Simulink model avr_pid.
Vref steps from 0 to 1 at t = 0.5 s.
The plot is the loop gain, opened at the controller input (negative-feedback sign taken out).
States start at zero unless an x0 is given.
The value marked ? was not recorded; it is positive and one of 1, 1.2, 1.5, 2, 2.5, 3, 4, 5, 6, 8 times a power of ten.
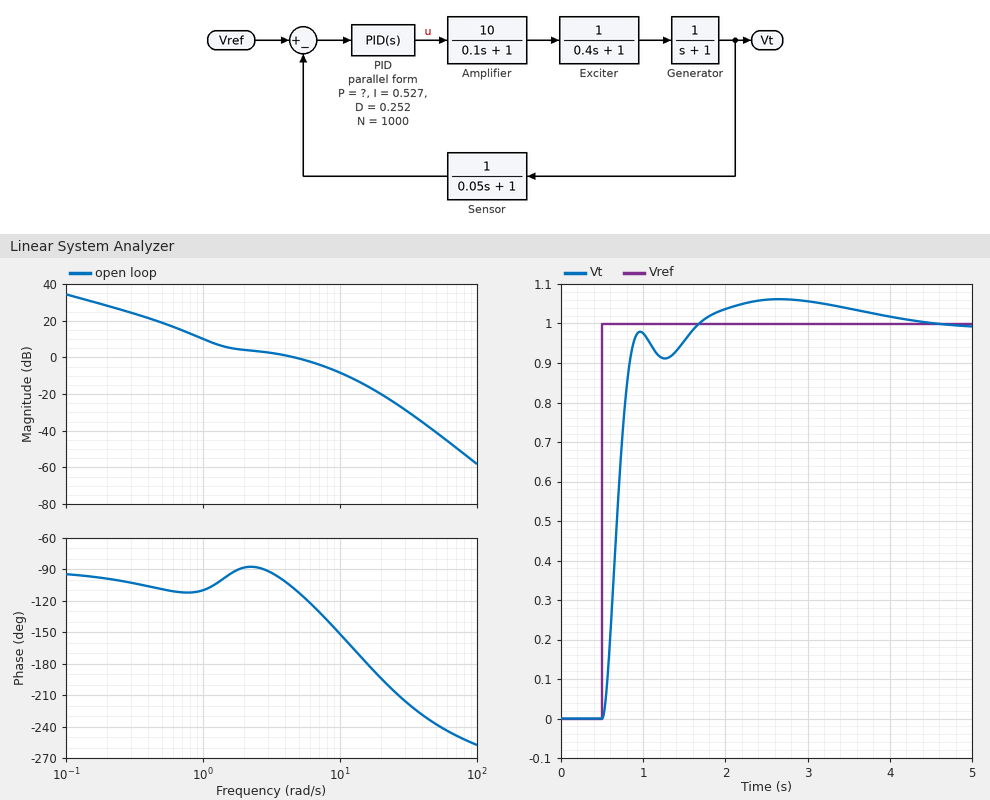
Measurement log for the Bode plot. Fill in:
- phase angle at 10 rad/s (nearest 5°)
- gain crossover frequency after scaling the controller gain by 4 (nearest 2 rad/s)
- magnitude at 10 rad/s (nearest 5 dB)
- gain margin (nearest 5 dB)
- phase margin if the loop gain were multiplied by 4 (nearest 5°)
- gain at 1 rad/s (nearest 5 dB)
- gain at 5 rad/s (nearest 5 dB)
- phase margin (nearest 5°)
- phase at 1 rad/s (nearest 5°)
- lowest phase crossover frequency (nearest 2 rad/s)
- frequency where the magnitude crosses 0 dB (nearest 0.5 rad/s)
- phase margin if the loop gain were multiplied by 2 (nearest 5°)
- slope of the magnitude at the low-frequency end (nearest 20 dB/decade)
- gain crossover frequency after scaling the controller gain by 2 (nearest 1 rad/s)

-150°
12 rad/s
-10 dB
15 dB
15°
10 dB
0 dB
70°
-110°
16 rad/s
4.5 rad/s
40°
-20 dB/decade
8 rad/s
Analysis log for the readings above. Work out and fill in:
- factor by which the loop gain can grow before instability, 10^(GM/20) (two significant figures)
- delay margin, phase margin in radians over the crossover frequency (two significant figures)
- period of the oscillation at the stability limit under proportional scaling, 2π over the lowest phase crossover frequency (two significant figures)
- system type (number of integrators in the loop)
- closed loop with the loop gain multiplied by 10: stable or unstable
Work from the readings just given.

5.6
0.27 s
0.39 s
1
unstable
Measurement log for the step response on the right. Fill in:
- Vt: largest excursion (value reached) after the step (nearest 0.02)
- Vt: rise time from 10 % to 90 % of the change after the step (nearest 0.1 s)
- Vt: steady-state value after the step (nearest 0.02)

1.06
0.3 s
1.00
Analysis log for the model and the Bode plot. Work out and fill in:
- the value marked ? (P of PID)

0.4
